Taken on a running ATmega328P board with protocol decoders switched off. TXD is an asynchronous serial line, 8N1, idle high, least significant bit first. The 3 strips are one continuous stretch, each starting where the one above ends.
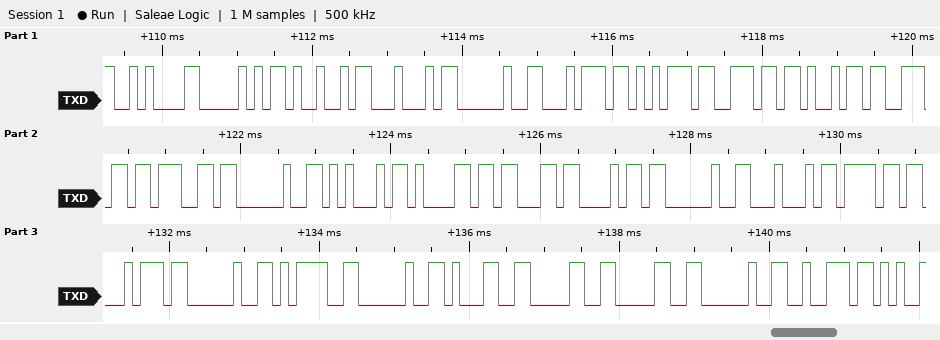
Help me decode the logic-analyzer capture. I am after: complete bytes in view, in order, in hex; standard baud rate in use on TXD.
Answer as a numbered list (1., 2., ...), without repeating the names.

1. 0A 50 49 44 20 74 75 6E 69 6E 67 20 45 61 63 68 20 44 6F 74 20 3D 20 31 30 30 20 72
2. 9600 baud
